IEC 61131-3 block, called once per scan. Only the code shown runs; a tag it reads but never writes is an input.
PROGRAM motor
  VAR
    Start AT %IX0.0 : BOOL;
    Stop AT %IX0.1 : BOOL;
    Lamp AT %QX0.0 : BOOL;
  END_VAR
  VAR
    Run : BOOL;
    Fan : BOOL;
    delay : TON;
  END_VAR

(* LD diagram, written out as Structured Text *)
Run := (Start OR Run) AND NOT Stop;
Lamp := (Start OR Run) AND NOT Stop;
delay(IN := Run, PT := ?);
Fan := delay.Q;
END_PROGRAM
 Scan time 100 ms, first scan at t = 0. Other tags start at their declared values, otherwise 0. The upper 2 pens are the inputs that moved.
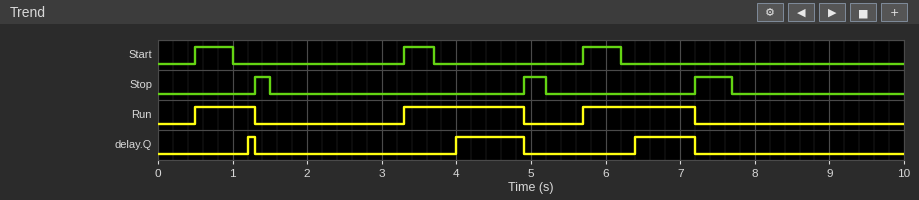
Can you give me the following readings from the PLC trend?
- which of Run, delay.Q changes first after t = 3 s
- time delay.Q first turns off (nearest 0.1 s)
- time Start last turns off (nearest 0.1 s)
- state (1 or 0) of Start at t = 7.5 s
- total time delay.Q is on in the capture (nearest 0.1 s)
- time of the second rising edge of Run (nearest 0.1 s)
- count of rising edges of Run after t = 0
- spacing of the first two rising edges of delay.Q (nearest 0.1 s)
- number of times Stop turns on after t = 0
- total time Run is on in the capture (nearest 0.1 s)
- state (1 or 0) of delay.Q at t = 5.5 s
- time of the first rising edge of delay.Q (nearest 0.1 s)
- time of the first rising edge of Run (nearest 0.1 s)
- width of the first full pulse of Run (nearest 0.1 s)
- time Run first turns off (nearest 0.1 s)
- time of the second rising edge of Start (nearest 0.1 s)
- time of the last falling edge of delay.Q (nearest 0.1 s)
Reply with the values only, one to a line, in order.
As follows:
Run
1.3 s
6.2 s
0
1.8 s
3.3 s
3
2.8 s
3
3.9 s
0
1.2 s
0.5 s
0.8 s
1.3 s
3.3 s
7.2 s
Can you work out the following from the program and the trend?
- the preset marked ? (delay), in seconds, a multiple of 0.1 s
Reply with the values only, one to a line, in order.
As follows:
0.7 s
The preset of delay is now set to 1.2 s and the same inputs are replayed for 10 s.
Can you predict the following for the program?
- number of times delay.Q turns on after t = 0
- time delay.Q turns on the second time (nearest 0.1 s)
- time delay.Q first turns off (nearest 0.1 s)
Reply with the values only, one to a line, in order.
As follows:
2
6.9 s
4.9 s
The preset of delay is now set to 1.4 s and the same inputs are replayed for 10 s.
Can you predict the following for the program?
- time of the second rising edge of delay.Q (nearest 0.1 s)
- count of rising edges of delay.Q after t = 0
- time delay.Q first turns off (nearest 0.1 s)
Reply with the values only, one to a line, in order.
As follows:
7.1 s
2
4.9 s
